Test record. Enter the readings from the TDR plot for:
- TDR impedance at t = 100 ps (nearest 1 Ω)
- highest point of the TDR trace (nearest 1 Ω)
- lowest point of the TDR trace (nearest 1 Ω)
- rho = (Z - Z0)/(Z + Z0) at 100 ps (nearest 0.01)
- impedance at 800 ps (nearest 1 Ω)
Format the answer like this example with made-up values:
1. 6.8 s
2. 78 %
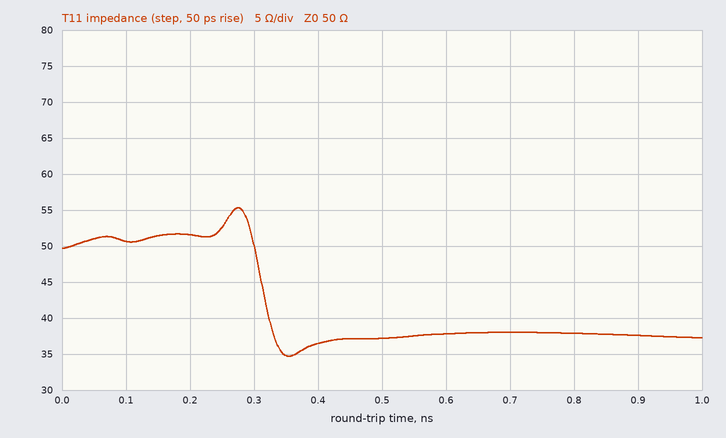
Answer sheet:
1. 51 Ω
2. 55 Ω
3. 35 Ω
4. +0.01
5. 38 Ω
